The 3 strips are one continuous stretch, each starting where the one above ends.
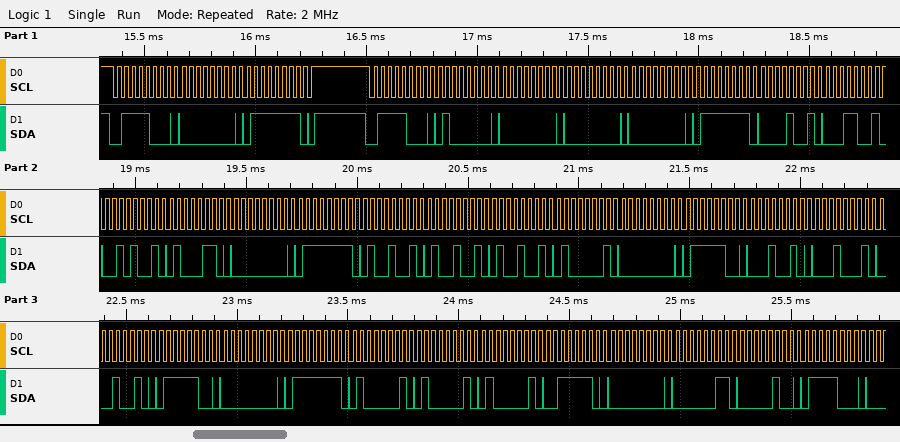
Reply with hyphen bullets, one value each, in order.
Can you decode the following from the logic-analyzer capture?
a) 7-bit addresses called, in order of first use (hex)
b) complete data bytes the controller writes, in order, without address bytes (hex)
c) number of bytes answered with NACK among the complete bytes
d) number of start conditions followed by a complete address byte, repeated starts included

- 0x3C
- 00 7F 40 00 00 00 7F 09 19 29 46 00 7F 49 49 49 41 00 7C 12 11 12 7C 00 7F 41 41 41 3E 00 03 04 78
- 0
- 2
